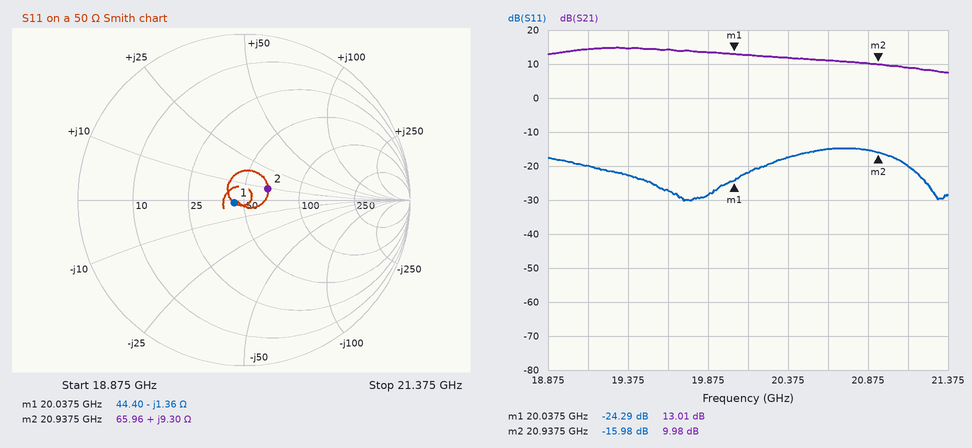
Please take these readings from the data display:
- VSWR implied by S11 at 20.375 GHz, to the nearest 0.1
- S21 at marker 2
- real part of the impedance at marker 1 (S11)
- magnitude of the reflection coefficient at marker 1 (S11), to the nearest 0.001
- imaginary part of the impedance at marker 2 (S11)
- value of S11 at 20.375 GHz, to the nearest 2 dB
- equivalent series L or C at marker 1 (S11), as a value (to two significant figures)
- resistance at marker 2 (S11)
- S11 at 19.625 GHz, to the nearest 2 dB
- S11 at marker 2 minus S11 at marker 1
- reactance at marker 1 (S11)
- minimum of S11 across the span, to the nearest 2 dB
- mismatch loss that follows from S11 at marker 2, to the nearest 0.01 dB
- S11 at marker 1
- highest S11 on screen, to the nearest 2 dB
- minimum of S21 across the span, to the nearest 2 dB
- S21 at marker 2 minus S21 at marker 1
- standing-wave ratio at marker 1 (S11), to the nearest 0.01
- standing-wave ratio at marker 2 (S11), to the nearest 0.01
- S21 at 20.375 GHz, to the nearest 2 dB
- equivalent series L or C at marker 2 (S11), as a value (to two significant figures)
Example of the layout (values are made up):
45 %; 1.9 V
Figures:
1.3; 9.98 dB; 44.40 Ω; 0.061; +9.30 Ω; -18 dB; 5.8 pF; 65.96 Ω; -28 dB; 8.31 dB; -1.36 Ω; -30 dB; 0.11 dB; -24.29 dB; -14 dB; 8 dB; -3.03 dB; 1.13; 1.38; 12 dB; 71 pH
